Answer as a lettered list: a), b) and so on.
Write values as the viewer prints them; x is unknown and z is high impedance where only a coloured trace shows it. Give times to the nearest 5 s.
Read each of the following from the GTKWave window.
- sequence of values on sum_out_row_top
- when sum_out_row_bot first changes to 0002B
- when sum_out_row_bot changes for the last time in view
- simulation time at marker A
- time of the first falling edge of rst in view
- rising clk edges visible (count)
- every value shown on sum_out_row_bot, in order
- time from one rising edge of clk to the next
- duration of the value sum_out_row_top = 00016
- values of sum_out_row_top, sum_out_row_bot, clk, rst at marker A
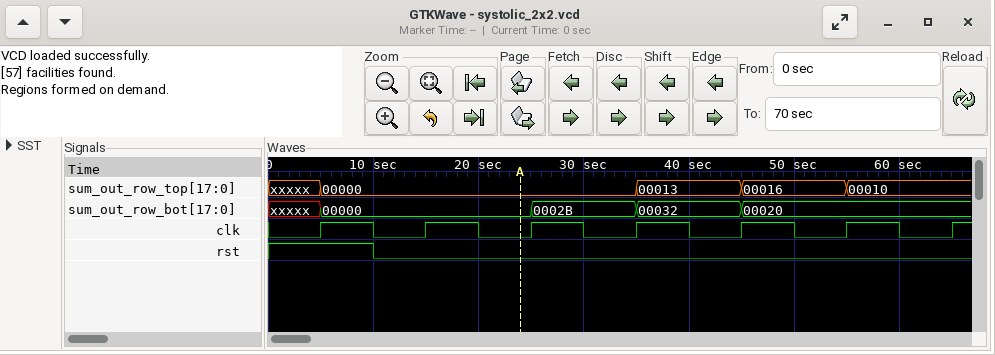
a) xxxxx, 00000, 00013, 00016, 00010
b) 25 s
c) 45 s
d) 25 s
e) 10 s
f) 7
g) xxxxx, 00000, 0002B, 00032, 00020
h) 10 s
i) 10 s
j) sum_out_row_top=00000, sum_out_row_bot=00000, clk=0, rst=0
